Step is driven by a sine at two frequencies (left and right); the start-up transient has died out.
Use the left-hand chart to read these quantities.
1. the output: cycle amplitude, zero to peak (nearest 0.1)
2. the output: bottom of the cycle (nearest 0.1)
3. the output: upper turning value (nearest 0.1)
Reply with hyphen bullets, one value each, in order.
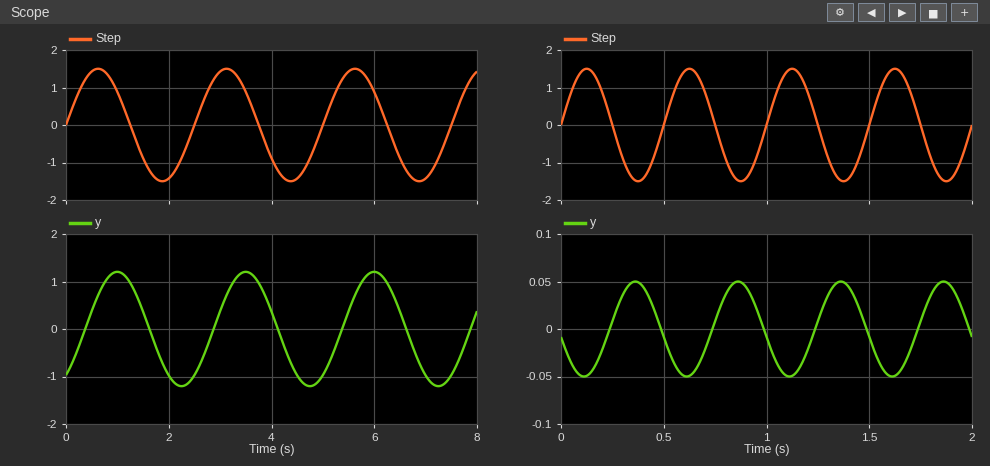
- 1.2
- -1.2
- 1.2
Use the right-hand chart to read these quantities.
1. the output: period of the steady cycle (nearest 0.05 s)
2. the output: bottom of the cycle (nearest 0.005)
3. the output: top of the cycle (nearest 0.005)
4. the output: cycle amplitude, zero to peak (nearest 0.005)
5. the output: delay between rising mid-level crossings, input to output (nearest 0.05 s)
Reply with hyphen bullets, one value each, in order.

- 0.50 s
- -0.050
- 0.050
- 0.050
- 0.25 s
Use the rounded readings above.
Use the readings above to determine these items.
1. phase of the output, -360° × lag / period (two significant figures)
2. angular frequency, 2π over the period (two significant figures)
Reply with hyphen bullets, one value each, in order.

- -180°
- 13 rad/s
